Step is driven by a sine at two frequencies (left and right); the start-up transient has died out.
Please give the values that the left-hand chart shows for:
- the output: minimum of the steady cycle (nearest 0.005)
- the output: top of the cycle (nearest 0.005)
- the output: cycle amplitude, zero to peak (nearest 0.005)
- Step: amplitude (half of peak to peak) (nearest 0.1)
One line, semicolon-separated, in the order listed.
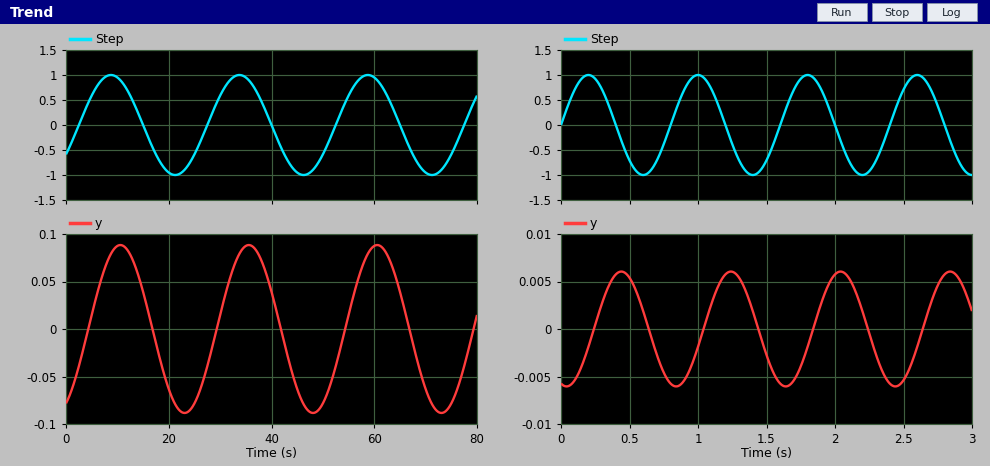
-0.090; 0.090; 0.090; 1.0
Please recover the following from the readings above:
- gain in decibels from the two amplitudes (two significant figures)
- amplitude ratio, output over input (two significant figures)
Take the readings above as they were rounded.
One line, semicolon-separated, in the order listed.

-21 dB; 0.090
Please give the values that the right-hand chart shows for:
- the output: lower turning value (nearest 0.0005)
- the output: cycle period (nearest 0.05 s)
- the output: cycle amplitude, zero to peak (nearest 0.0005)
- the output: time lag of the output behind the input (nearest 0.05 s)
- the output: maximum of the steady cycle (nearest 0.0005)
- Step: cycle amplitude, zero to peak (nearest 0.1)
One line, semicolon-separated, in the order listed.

-0.0060; 0.80 s; 0.0060; 0.25 s; 0.0060; 1.0
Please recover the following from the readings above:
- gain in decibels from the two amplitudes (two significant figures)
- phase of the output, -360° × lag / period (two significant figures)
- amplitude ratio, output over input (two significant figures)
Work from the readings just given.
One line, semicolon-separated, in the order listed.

-44 dB; -110°; 0.0060
